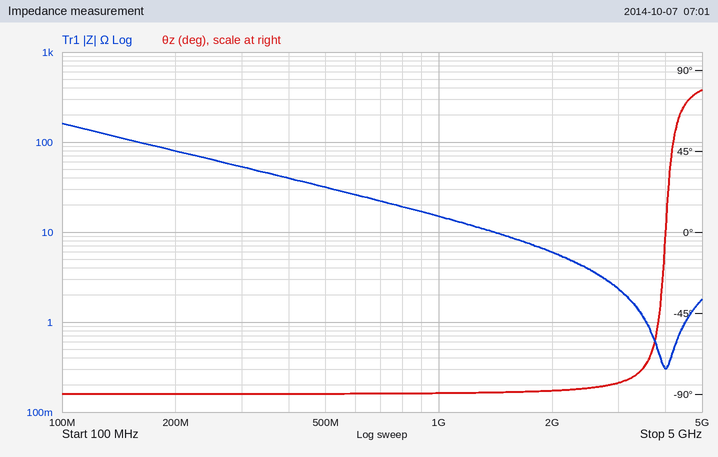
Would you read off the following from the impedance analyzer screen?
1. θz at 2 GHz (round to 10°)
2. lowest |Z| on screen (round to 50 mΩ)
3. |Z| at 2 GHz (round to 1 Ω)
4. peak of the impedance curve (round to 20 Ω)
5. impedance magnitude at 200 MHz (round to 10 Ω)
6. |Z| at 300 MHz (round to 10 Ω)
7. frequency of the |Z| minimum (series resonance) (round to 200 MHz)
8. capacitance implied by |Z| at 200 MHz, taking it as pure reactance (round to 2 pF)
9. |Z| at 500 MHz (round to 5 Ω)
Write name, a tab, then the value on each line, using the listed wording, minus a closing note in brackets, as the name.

θz at 2 GHz	-90°
lowest |Z| on screen	300 mΩ
|Z| at 2 GHz	6 Ω
peak of the impedance curve	160 Ω
impedance magnitude at 200 MHz	80 Ω
|Z| at 300 MHz	50 Ω
frequency of the |Z| minimum (series resonance)	4.0 GHz
capacitance implied by |Z| at 200 MHz, taking it as pure reactance	10 pF
|Z| at 500 MHz	30 Ω
